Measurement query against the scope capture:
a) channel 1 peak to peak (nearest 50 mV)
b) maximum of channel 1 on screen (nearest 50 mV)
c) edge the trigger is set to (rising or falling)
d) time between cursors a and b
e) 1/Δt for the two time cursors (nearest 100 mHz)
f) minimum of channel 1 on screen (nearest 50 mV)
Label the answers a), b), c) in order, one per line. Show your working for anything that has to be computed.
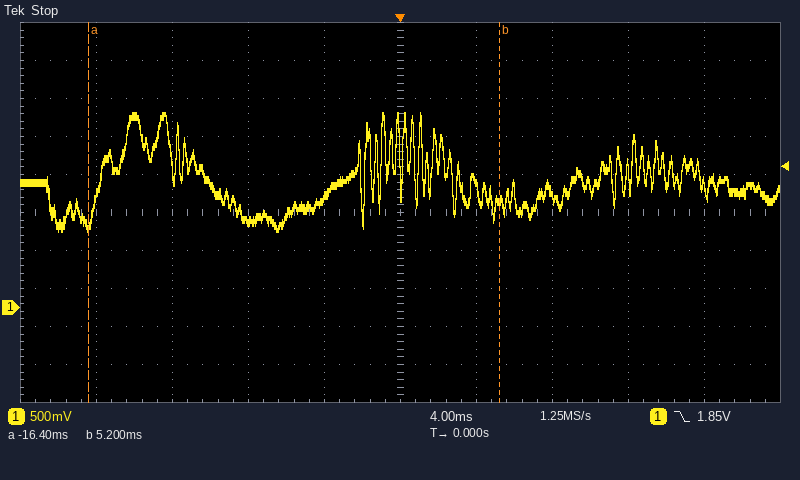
a) 2.55 V − (1.00 V) = 1.55 V
b) 2.55 V
c) falling
d) 5.2 ms − (-16.4 ms) = 21.6 ms
e) 1 / 21.6 ms ≈ 46.3 Hz
f) 1.00 V
